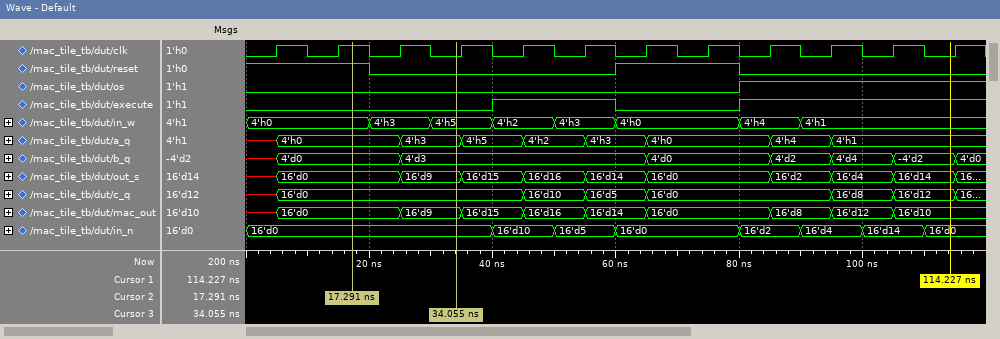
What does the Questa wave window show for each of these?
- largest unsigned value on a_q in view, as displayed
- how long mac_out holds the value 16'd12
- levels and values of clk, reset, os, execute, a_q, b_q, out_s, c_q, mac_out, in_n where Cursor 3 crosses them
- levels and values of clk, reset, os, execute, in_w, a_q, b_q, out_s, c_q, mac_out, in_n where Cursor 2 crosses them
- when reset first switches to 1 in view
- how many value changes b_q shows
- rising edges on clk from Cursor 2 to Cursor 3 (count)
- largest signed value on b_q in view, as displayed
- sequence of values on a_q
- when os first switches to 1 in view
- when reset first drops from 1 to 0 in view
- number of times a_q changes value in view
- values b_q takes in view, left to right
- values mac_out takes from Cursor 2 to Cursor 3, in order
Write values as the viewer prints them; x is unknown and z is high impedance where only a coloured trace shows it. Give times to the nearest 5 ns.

4'h5
10 ns
clk=0, reset=0, os=0, execute=0, a_q=4'h3, b_q=4'd3, out_s=16'd9, c_q=16'd0, mac_out=16'd9, in_n=16'd0
clk=1, reset=1, os=0, execute=0, in_w=4'h0, a_q=4'h0, b_q=4'd0, out_s=16'd0, c_q=16'd0, mac_out=16'd0, in_n=16'd0
60 ns
7
1
4'd4
x, 4'h0, 4'h3, 4'h5, 4'h2, 4'h3, 4'h0, 4'h4, 4'h1
80 ns
20 ns
8
x, 4'd0, 4'd3, 4'd0, 4'd2, 4'd4, -4'd2, 4'd0
16'd0, 16'd9
